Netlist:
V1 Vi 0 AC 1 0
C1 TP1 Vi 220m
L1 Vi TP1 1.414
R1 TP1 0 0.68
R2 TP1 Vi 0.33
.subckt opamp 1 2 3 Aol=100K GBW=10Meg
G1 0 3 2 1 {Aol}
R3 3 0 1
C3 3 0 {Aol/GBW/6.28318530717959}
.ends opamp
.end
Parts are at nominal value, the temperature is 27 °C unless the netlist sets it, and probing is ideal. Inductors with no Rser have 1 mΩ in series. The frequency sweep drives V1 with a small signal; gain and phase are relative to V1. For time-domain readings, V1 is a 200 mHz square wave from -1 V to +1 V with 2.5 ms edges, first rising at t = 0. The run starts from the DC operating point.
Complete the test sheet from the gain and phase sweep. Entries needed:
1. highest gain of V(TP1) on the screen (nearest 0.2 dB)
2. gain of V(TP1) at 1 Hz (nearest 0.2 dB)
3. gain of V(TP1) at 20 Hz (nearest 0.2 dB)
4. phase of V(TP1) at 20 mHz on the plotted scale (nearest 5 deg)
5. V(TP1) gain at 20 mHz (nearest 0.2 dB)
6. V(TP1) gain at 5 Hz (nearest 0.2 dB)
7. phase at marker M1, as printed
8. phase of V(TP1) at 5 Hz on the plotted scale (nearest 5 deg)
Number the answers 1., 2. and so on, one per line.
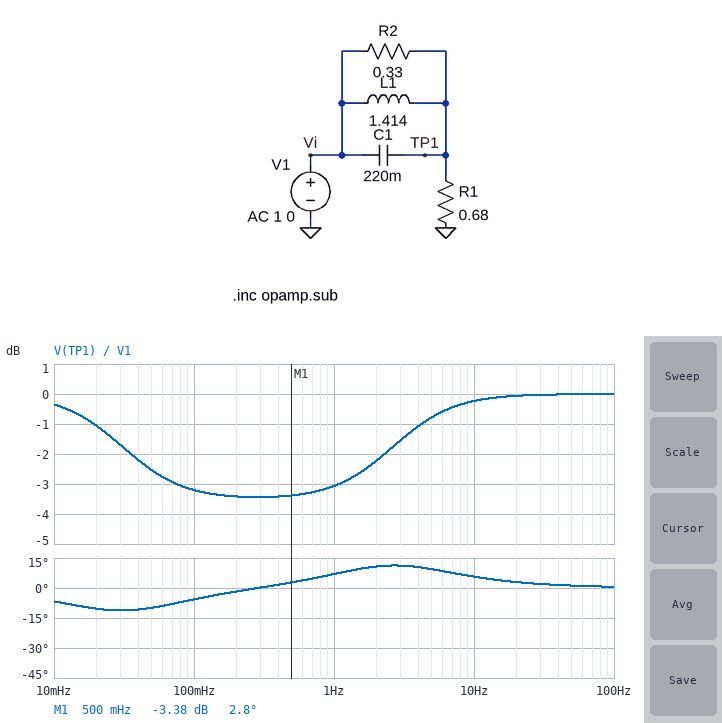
1. 0 dB
2. -3.0 dB
3. 0 dB
4. -10 deg
5. -1.0 dB
6. -0.8 dB
7. 2.8 deg
8. 10 deg
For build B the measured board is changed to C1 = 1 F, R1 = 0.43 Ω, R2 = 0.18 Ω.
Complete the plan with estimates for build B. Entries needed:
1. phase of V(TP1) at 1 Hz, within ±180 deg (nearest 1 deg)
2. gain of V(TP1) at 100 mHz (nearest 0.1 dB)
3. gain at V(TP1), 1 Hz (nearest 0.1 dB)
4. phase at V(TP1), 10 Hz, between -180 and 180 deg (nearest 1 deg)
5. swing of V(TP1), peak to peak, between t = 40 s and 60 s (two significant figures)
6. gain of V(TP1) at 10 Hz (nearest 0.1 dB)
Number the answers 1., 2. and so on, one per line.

1. 10 deg
2. -3.0 dB
3. -1.6 dB
4. 2 deg
5. 2.5 V
6. 0 dB
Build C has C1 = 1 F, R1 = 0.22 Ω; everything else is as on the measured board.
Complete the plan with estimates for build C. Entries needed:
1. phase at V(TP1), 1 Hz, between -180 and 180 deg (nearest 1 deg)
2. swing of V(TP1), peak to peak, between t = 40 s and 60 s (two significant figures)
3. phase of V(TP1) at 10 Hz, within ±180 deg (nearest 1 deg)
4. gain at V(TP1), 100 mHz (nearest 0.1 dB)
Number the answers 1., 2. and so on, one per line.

1. 25 deg
2. 3.1 V
3. 4 deg
4. -7.9 dB
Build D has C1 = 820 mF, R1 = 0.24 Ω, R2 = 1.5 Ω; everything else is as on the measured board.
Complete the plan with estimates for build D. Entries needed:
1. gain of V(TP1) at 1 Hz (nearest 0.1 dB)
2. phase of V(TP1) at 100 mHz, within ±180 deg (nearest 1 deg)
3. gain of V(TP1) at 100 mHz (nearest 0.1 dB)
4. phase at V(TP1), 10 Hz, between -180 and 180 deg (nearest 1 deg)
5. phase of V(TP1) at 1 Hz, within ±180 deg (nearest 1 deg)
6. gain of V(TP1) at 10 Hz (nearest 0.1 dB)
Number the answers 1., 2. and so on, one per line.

1. -2.8 dB
2. -35 deg
3. -14.6 dB
4. 5 deg
5. 36 deg
6. 0 dB
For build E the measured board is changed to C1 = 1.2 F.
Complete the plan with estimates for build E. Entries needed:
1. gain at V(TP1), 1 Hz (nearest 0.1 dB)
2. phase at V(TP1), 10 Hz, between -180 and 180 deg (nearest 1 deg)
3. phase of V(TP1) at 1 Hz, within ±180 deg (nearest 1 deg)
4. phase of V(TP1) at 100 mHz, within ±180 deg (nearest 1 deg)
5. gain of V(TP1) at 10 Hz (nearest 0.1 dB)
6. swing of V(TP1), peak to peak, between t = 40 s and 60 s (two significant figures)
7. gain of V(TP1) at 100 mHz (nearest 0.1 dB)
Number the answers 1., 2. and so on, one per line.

1. -0.7 dB
2. 1 deg
3. 9 deg
4. -2 deg
5. 0 dB
6. 2.6 V
7. -3.4 dB
